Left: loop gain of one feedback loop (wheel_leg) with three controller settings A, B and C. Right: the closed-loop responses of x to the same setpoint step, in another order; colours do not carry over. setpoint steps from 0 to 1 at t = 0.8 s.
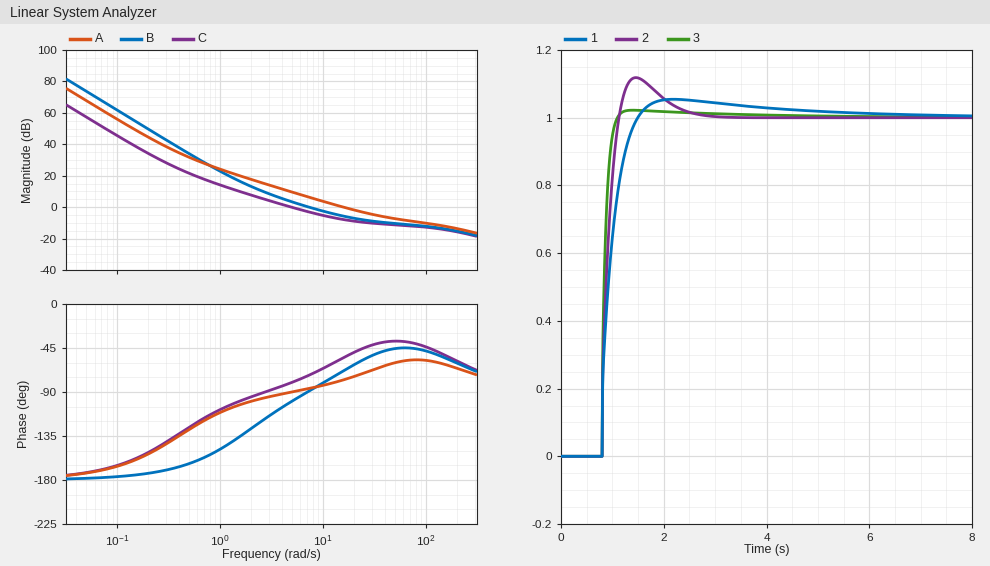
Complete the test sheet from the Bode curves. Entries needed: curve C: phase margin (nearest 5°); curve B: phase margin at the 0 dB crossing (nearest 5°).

100°
90°
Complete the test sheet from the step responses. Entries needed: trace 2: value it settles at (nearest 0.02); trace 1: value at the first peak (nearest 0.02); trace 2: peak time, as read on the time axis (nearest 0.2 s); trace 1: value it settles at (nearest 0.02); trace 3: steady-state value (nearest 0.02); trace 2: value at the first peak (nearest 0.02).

1.00
1.06
1.4 s
1.00
1.00
1.12
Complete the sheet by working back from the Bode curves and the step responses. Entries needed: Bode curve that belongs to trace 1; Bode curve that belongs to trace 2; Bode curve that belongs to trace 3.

C
B
A
